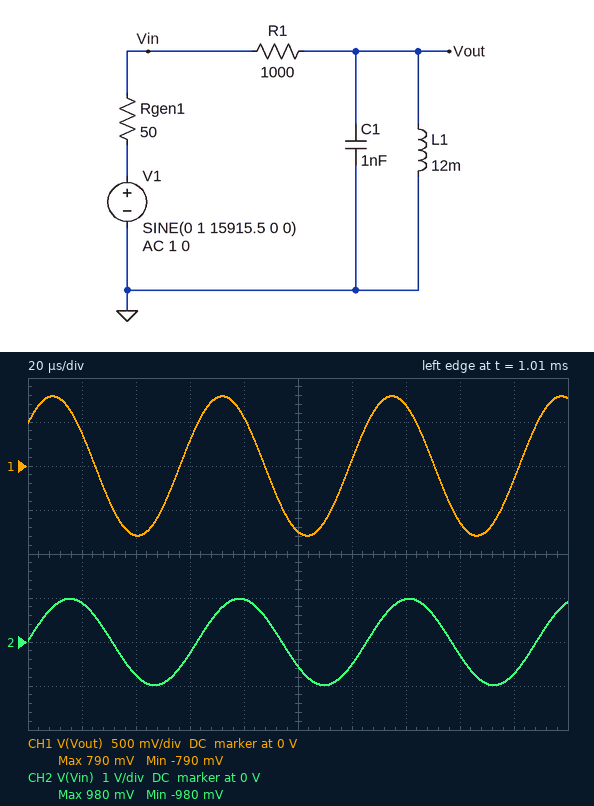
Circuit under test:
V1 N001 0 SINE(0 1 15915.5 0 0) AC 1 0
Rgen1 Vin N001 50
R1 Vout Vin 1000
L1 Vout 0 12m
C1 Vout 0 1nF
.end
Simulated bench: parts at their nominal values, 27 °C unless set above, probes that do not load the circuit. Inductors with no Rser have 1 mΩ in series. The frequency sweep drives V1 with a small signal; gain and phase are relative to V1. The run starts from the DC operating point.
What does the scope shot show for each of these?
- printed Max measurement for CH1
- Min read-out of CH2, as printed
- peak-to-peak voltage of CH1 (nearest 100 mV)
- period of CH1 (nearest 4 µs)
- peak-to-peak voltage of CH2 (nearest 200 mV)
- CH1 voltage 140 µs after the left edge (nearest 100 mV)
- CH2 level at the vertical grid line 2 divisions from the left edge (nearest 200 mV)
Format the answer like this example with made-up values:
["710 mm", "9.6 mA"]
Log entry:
["790 mV", "-980 mV", "1.6 V", "64 µs", "2.0 V", "700 mV", "-800 mV"]
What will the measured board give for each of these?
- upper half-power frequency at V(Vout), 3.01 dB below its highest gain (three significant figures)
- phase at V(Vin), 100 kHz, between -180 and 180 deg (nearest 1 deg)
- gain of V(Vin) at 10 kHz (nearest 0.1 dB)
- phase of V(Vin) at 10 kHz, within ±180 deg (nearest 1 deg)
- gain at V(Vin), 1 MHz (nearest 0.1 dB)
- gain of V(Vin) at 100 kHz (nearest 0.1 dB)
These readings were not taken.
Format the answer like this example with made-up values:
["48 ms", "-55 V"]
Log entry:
["164 kHz", "-1 deg", "-0.3 dB", "1 deg", "-0.4 dB", "-0.1 dB"]
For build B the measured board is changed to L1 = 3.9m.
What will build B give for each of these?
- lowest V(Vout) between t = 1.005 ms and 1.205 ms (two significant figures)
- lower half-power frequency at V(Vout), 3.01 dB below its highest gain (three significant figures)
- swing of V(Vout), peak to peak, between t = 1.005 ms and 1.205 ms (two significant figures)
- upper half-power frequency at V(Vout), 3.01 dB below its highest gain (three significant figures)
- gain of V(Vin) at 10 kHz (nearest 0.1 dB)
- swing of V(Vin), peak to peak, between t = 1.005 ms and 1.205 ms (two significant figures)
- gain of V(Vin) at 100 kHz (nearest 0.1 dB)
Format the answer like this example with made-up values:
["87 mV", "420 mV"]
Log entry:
["-360 mV", "34.8 kHz", "720 mV", "186 kHz", "-0.4 dB", "1.9 V", "0 dB"]
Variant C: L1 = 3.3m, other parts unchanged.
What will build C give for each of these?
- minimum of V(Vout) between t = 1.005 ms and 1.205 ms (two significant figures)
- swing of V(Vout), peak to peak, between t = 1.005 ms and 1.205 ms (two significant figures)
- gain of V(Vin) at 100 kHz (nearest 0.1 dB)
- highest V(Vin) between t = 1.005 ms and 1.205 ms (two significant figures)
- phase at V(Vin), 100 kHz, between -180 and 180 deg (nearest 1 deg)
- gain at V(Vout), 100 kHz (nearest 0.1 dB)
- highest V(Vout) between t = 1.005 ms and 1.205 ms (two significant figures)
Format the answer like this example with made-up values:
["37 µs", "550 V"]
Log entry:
["-310 mV", "620 mV", "0 dB", "960 mV", "0 deg", "-0.1 dB", "310 mV"]
